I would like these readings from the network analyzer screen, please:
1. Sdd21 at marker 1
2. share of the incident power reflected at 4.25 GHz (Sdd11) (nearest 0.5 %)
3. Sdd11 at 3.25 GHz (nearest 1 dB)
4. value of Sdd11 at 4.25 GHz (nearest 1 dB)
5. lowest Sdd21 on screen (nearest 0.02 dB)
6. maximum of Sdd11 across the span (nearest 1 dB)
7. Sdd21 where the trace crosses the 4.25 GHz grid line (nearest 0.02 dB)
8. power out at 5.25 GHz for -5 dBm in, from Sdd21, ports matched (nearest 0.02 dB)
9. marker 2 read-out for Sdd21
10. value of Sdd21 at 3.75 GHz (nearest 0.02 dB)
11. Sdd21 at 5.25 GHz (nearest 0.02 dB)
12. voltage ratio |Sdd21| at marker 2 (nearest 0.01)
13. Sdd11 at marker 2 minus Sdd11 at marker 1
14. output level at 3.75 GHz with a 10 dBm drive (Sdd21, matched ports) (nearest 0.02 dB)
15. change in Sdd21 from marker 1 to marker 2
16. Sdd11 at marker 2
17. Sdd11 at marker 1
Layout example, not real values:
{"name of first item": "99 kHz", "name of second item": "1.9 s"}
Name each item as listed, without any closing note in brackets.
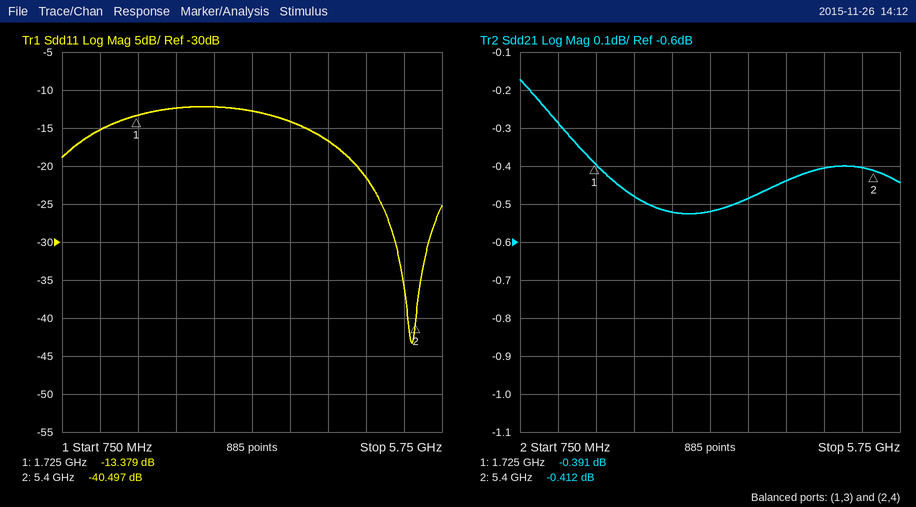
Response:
{"Sdd21 at marker 1": "-0.391 dB", "share of the incident power reflected at 4.25 GHz (Sdd11)": "2.0 %", "Sdd11 at 3.25 GHz": "-13 dB", "value of Sdd11 at 4.25 GHz": "-17 dB", "lowest Sdd21 on screen": "-0.52 dB", "maximum of Sdd11 across the span": "-12 dB", "Sdd21 where the trace crosses the 4.25 GHz grid line": "-0.44 dB", "power out at 5.25 GHz for -5 dBm in, from Sdd21, ports matched": "-5.40 dBm", "marker 2 read-out for Sdd21": "-0.412 dB", "value of Sdd21 at 3.75 GHz": "-0.48 dB", "Sdd21 at 5.25 GHz": "-0.40 dB", "voltage ratio |Sdd21| at marker 2": "0.95", "Sdd11 at marker 2 minus Sdd11 at marker 1": "-27.118 dB", "output level at 3.75 GHz with a 10 dBm drive (Sdd21, matched ports)": "9.52 dBm", "change in Sdd21 from marker 1 to marker 2": "-0.021 dB", "Sdd11 at marker 2": "-40.497 dB", "Sdd11 at marker 1": "-13.379 dB"}
